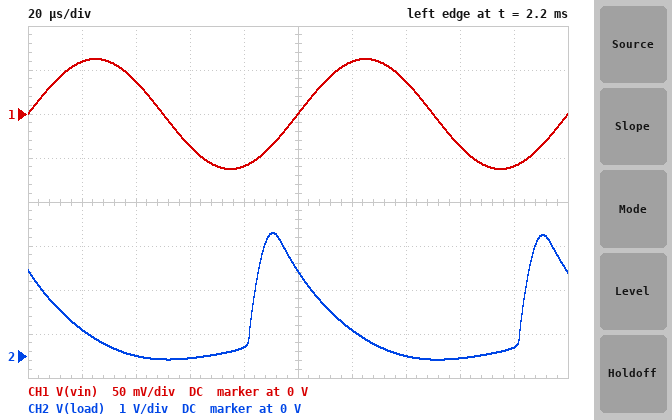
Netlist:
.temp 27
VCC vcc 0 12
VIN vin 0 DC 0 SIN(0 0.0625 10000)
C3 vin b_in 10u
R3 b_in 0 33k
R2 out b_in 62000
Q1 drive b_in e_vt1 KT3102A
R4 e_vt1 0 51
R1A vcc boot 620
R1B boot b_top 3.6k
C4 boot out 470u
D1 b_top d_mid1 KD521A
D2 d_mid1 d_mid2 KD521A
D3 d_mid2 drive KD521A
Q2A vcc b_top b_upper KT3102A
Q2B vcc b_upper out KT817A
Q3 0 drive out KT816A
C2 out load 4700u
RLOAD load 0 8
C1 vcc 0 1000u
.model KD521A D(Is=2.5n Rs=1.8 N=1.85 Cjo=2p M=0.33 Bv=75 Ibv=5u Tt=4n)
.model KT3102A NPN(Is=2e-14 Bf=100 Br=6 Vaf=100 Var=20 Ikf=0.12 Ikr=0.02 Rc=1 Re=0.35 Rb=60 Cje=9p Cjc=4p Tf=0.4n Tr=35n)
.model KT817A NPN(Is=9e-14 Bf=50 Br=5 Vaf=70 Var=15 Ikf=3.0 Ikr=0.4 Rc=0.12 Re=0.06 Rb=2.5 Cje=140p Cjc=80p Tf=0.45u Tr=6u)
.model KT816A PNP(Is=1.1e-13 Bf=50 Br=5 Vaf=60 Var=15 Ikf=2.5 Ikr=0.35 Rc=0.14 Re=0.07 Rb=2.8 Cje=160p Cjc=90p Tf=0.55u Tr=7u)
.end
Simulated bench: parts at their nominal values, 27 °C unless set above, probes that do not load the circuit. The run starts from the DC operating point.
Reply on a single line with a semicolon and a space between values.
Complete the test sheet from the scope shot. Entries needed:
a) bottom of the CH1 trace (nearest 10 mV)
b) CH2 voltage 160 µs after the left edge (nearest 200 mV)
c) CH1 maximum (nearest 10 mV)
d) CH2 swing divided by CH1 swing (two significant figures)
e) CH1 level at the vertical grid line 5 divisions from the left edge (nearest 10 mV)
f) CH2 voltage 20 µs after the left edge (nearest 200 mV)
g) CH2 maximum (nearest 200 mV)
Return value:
-60 mV; 0 V; 60 mV; 23; 0 V; 600 mV; 2.8 V
